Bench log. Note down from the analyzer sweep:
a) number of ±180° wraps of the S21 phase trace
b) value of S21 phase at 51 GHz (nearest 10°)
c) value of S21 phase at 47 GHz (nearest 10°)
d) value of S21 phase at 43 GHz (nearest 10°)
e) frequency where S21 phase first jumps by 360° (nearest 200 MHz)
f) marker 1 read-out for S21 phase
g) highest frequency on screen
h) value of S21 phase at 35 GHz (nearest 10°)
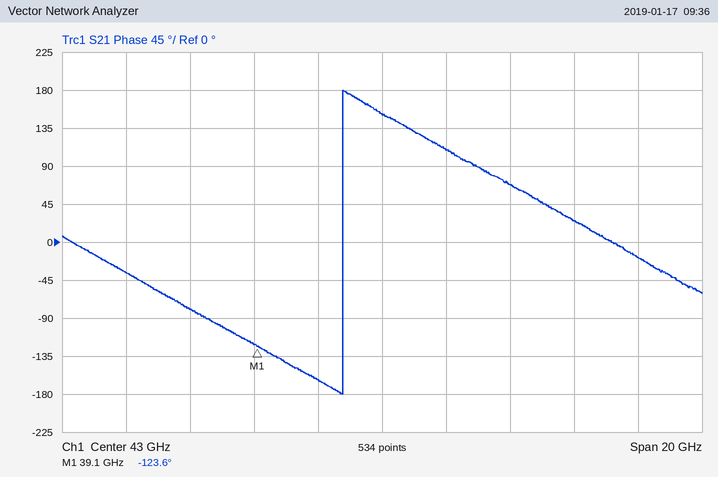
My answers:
1
-20°
70°
150°
41.8 GHz
-123.6°
53 GHz
-40°
